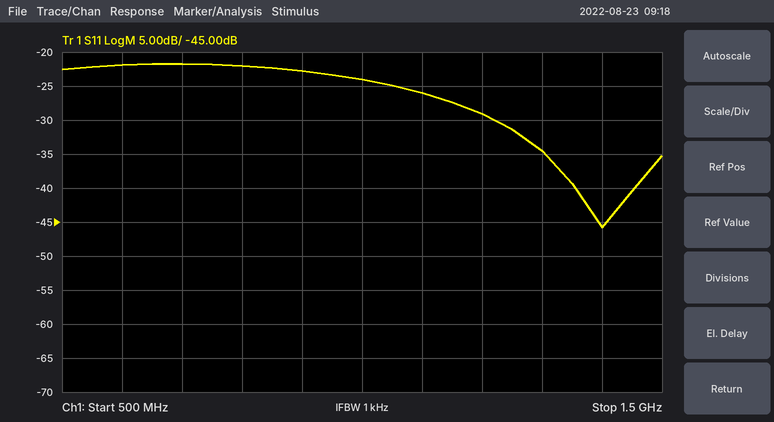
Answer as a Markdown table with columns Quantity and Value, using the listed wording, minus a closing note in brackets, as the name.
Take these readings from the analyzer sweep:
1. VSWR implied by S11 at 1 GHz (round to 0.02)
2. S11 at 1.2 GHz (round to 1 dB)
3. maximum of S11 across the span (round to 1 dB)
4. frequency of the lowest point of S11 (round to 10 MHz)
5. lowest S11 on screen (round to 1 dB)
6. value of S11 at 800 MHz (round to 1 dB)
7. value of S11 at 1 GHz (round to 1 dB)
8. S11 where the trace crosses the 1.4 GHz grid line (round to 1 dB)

| Quantity | Value |
|---|---|
| VSWR implied by S11 at 1 GHz | 1.14 |
| S11 at 1.2 GHz | -29 dB |
| maximum of S11 across the span | -22 dB |
| frequency of the lowest point of S11 | 1.40 GHz |
| lowest S11 on screen | -46 dB |
| value of S11 at 800 MHz | -22 dB |
| value of S11 at 1 GHz | -24 dB |
| S11 where the trace crosses the 1.4 GHz grid line | -46 dB |
